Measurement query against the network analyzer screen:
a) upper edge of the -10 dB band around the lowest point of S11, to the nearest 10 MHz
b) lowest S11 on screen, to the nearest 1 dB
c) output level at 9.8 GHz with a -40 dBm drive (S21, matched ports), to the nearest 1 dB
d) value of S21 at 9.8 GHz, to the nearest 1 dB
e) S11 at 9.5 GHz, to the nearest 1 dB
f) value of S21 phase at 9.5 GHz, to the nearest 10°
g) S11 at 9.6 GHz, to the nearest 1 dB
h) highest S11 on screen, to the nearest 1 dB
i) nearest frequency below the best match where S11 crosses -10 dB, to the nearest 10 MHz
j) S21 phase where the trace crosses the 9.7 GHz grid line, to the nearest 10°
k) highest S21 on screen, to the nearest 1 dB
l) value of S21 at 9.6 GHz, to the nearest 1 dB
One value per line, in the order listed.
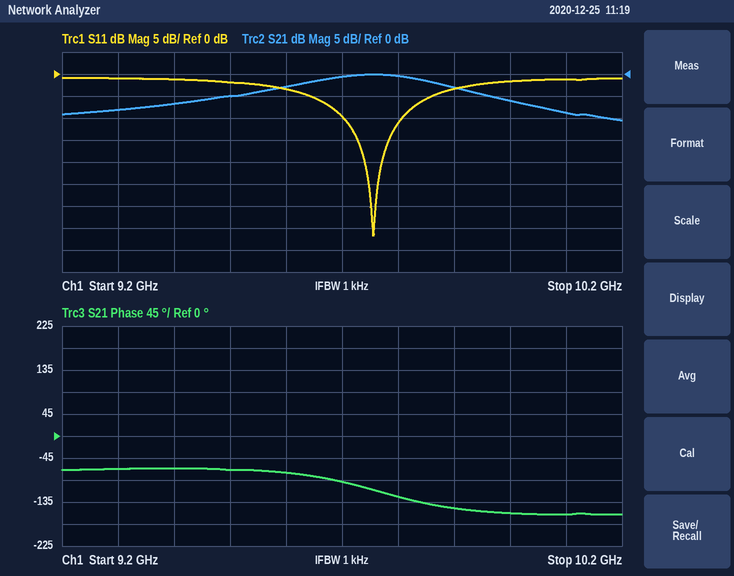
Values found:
9.81 GHz
-37 dB
-40 dBm
0 dB
-2 dB
-70°
-3 dB
-1 dB
9.70 GHz
-90°
0 dB
-3 dB
